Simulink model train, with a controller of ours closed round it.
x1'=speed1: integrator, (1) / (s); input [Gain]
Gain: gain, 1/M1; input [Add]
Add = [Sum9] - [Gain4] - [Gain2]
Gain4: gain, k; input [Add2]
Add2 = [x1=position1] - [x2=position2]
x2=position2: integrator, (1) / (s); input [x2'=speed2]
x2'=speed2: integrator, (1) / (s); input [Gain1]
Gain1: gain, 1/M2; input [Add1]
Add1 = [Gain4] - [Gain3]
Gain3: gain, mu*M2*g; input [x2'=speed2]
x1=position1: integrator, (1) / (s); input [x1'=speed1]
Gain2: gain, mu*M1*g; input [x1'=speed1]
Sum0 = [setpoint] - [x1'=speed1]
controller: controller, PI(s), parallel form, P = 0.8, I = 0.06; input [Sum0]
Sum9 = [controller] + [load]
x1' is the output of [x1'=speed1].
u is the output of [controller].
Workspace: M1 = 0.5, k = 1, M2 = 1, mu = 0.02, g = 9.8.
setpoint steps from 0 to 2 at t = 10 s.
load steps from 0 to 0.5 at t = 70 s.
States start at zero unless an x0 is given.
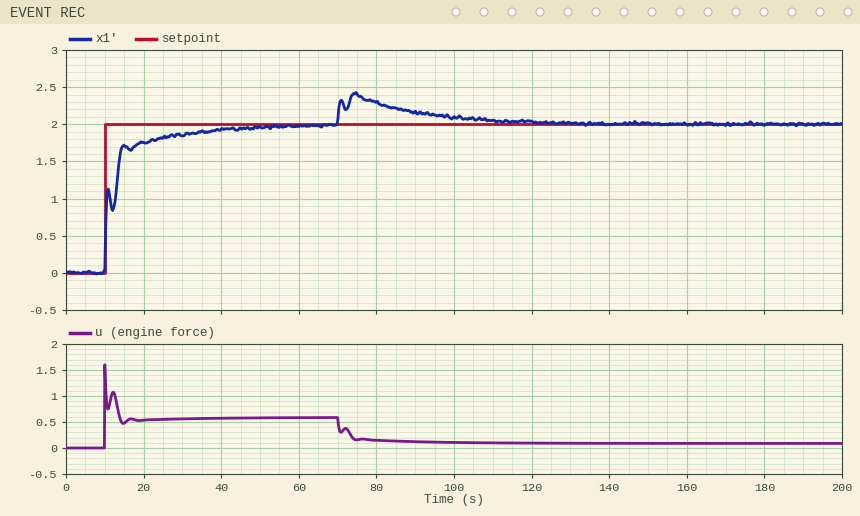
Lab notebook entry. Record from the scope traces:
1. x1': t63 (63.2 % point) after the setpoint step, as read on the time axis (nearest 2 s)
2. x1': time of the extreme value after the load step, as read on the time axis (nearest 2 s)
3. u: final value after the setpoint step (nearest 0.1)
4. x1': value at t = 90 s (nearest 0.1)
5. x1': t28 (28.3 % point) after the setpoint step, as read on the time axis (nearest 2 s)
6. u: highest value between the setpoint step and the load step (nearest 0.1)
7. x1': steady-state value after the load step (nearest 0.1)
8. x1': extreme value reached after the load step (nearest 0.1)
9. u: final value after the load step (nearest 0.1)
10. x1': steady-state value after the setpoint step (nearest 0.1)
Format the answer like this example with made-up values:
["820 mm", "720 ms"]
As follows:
["14 s", "74 s", "0.6", "2.2", "10 s", "1.6", "2.0", "2.4", "0.1", "2.0"]
